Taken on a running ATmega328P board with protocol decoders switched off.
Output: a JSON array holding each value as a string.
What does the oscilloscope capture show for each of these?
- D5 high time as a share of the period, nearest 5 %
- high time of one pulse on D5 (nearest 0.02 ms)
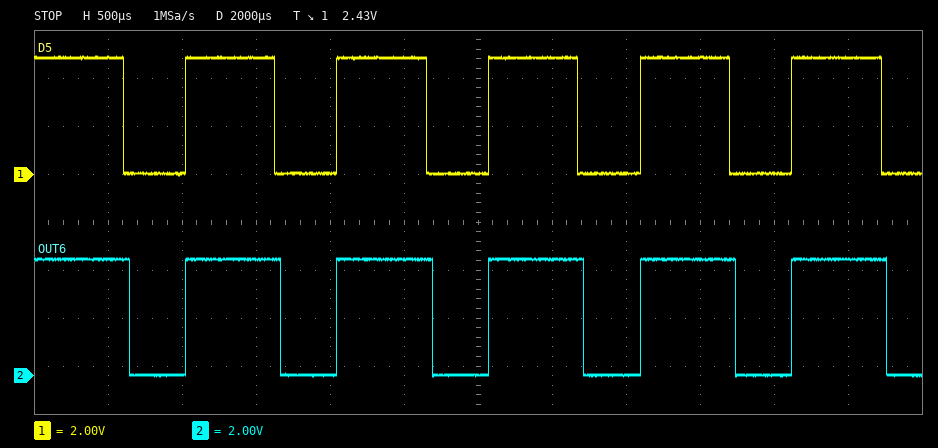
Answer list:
["60 %", "0.60 ms"]
